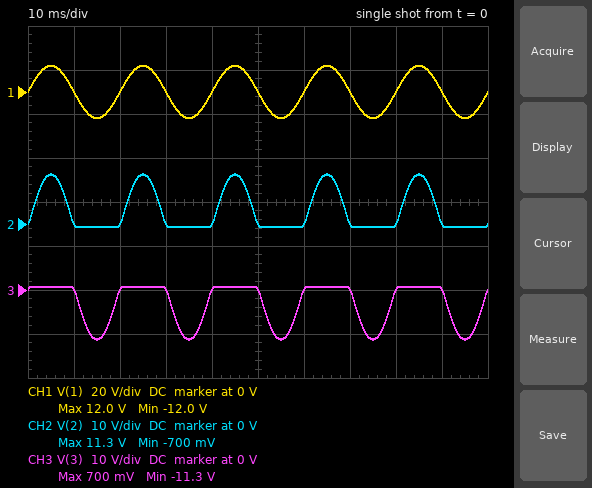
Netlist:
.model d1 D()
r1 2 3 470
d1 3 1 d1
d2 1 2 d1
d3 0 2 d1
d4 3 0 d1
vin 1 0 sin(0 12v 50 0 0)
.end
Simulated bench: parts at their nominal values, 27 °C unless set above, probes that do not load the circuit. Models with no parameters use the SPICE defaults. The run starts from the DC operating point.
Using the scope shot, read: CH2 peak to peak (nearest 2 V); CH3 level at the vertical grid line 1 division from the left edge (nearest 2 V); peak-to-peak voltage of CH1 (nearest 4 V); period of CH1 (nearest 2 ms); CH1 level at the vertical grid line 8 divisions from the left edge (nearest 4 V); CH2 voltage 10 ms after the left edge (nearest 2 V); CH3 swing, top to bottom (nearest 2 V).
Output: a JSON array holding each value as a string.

["12 V", "0 V", "24 V", "20 ms", "0 V", "0 V", "12 V"]
